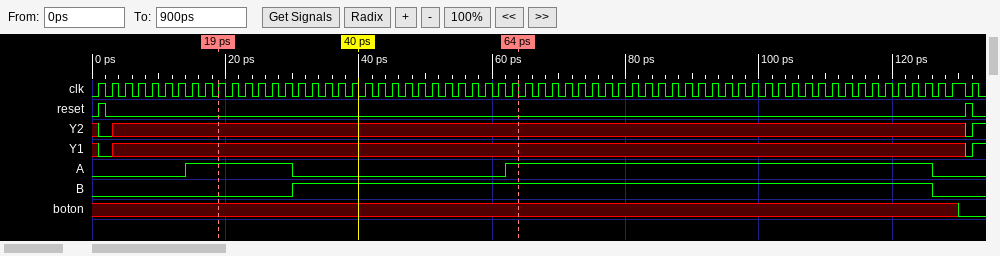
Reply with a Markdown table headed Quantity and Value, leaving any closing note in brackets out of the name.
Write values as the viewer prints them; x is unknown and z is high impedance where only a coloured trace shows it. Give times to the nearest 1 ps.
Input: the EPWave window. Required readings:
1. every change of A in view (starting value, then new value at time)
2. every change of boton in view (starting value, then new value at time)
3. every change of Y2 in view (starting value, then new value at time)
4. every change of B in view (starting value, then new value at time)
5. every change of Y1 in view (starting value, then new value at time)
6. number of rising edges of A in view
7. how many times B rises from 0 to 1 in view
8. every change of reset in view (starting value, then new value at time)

| Quantity | Value |
|---|---|
| every change of A in view | 0, 1 at 14 ps, 0 at 30 ps, 1 at 62 ps, 0 at 126 ps |
| every change of boton in view | x, 0 at 130 ps |
| every change of Y2 in view | x, 0 at 1 ps, x at 3 ps, 0 at 131 ps, 1 at 132 ps |
| every change of B in view | 0, 1 at 30 ps, 0 at 126 ps |
| every change of Y1 in view | x, 0 at 1 ps, x at 3 ps, 0 at 131 ps, 1 at 132 ps |
| number of rising edges of A in view | 2 |
| how many times B rises from 0 to 1 in view | 1 |
| every change of reset in view | 0, 1 at 1 ps, 0 at 2 ps, 1 at 131 ps, 0 at 132 ps |
